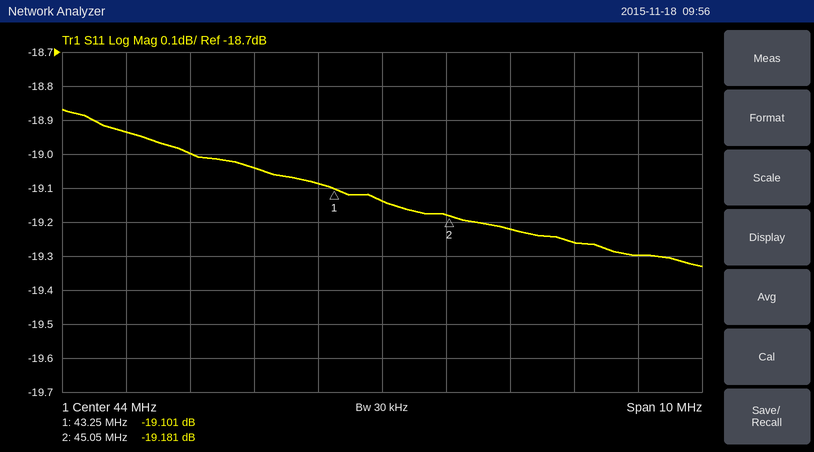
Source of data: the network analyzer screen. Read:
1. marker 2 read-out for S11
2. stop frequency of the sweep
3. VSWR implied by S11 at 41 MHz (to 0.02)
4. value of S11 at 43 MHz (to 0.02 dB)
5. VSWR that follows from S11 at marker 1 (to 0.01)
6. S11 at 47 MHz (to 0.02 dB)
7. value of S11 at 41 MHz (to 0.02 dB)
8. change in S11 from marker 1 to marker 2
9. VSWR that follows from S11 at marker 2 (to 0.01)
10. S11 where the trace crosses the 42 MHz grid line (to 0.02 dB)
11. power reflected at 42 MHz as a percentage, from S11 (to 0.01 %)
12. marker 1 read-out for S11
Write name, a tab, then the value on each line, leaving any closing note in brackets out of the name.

marker 2 read-out for S11	-19.181 dB
stop frequency of the sweep	49 MHz
VSWR implied by S11 at 41 MHz	1.26
value of S11 at 43 MHz	-19.08 dB
VSWR that follows from S11 at marker 1	1.25
S11 at 47 MHz	-19.26 dB
value of S11 at 41 MHz	-19.00 dB
change in S11 from marker 1 to marker 2	-0.080 dB
VSWR that follows from S11 at marker 2	1.25
S11 where the trace crosses the 42 MHz grid line	-19.04 dB
power reflected at 42 MHz as a percentage, from S11	1.25 %
marker 1 read-out for S11	-19.101 dB
